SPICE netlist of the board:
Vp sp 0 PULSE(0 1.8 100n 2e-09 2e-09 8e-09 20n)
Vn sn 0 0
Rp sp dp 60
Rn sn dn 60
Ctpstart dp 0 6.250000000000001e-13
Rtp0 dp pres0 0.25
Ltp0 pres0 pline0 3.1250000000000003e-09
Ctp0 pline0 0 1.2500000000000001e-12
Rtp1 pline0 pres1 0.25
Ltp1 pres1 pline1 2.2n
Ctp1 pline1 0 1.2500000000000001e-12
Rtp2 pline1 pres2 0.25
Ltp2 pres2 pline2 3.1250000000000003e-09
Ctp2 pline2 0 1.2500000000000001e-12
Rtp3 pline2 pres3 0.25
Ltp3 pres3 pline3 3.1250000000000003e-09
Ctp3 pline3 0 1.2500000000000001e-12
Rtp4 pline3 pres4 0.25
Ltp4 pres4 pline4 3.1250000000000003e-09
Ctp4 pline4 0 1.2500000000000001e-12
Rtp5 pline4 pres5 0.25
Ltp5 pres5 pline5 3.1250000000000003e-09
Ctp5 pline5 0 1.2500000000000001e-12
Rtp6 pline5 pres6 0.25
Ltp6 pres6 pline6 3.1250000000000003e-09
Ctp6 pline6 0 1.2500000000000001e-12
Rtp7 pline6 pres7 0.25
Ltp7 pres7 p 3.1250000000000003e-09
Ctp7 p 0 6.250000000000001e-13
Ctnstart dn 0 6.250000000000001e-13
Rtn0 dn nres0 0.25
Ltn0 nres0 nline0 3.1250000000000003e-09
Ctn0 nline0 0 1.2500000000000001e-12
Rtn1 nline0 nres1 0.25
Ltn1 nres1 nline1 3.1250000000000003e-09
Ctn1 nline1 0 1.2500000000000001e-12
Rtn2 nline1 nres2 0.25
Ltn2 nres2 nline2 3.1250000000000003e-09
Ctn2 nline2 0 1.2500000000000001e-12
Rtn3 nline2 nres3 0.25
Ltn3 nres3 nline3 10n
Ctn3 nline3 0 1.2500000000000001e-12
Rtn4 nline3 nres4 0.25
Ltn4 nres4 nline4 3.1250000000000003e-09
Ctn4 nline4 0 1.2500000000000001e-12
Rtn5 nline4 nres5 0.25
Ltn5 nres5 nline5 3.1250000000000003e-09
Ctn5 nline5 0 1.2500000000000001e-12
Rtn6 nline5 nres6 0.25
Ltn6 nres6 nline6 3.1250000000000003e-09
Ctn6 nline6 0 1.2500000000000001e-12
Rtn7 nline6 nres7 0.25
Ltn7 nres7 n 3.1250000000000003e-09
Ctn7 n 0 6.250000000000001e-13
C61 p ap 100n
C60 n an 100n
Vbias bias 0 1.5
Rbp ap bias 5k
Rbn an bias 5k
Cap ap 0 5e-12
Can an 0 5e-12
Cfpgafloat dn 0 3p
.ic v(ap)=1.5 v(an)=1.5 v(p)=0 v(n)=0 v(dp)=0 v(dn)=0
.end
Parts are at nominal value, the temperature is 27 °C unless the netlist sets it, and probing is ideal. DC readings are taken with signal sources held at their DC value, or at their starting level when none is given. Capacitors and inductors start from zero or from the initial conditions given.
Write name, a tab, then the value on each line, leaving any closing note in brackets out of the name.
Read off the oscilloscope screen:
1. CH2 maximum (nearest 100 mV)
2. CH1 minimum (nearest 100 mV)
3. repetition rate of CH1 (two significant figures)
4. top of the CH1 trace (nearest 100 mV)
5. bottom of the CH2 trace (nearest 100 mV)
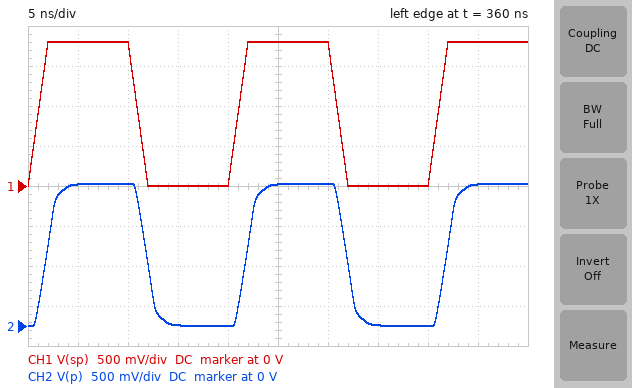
CH2 maximum	1.8 V
CH1 minimum	0 V
repetition rate of CH1	50 MHz
top of the CH1 trace	1.8 V
bottom of the CH2 trace	0 V
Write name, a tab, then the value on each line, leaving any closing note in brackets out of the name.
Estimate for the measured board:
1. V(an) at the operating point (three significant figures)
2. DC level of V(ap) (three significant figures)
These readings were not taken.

V(an) at the operating point	1.50 V
DC level of V(ap)	1.50 V
